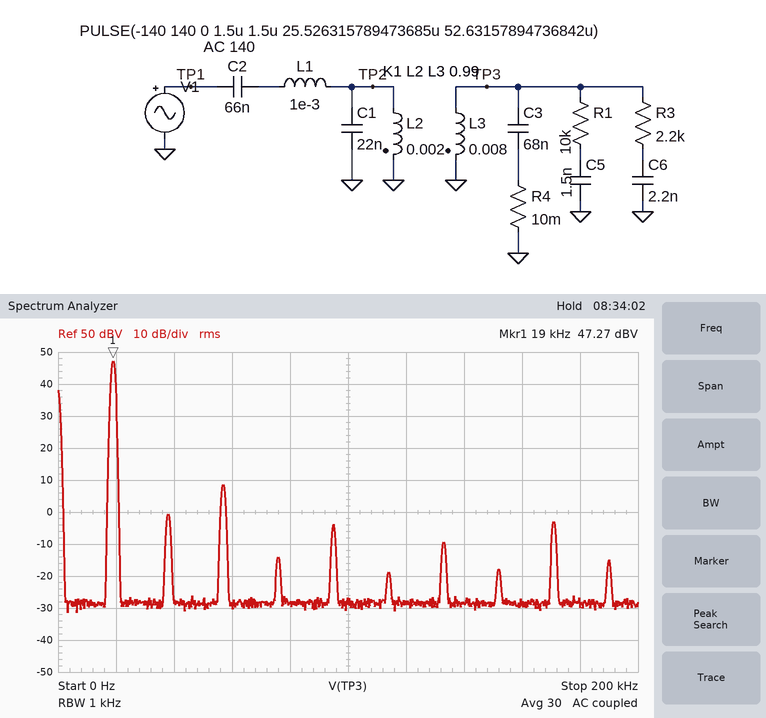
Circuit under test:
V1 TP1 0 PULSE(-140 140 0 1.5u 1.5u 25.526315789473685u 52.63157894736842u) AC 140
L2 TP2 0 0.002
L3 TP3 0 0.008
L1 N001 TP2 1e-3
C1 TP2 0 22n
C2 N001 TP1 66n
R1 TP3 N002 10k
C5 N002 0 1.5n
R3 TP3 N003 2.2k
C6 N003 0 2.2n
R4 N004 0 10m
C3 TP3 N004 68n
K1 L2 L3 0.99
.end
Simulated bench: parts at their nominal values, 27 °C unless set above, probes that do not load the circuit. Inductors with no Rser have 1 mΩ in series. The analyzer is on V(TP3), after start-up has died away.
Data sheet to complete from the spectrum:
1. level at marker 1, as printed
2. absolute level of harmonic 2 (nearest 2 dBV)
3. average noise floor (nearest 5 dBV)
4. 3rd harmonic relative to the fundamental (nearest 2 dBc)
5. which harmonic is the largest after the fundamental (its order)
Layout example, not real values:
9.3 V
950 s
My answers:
47.27 dBV
0 dBV
-30 dBV
-38 dBc
3
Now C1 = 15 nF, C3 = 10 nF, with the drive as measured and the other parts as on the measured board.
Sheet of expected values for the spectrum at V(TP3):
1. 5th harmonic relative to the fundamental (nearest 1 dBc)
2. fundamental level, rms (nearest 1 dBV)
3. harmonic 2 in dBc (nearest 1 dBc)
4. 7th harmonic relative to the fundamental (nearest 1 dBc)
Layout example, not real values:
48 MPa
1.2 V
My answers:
-38 dBc
48 dBV
-29 dBc
-46 dBc
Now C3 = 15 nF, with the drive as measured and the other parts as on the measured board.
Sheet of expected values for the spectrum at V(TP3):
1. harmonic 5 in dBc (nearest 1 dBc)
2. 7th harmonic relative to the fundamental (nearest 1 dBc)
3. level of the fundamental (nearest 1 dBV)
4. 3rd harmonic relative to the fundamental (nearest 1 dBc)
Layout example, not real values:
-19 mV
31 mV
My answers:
-41 dBc
-48 dBc
48 dBV
-27 dBc
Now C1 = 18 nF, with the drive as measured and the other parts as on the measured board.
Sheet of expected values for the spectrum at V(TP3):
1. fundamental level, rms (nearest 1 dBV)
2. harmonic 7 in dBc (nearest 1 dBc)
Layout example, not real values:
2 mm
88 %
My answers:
47 dBV
-58 dBc
